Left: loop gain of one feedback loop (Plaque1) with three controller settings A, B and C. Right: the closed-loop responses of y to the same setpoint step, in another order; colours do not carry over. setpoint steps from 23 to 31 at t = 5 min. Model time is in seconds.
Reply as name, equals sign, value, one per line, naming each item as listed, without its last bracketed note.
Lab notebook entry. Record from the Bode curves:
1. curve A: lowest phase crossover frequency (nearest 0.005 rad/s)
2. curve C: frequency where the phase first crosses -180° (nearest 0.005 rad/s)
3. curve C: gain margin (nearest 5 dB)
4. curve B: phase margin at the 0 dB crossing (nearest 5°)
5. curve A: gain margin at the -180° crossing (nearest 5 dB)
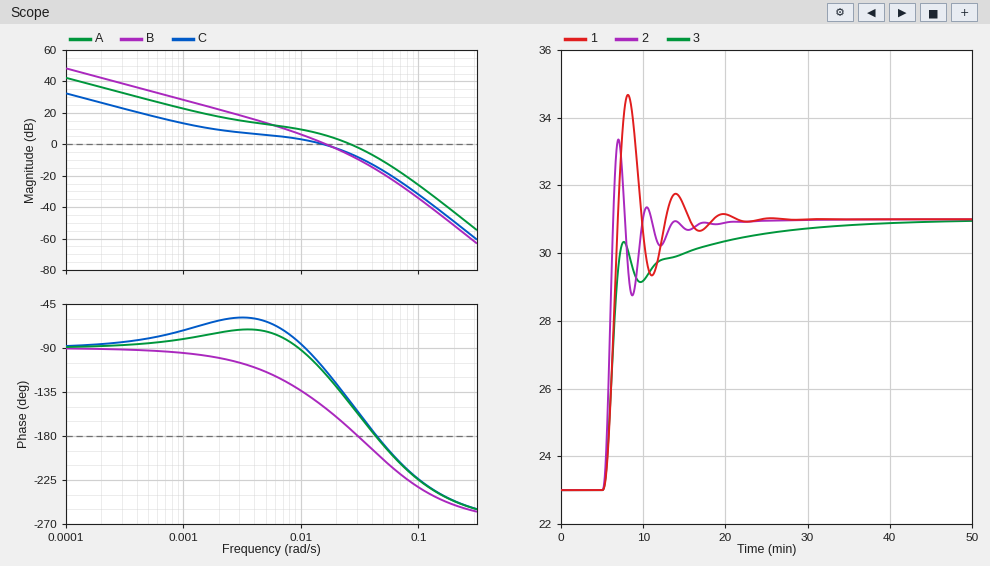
curve A: lowest phase crossover frequency = 0.045 rad/s
curve C: frequency where the phase first crosses -180° = 0.045 rad/s
curve C: gain margin = 15 dB
curve B: phase margin at the 0 dB crossing = 30°
curve A: gain margin at the -180° crossing = 10 dB
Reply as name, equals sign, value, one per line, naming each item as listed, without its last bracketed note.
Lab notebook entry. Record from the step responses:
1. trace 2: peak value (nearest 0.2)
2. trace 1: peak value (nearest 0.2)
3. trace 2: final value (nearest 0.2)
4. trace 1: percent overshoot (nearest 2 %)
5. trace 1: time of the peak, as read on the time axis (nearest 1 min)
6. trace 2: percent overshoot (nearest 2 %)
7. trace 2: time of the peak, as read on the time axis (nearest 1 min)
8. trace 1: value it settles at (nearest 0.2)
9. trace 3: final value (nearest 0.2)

trace 2: peak value = 33.4
trace 1: peak value = 34.6
trace 2: final value = 31.0
trace 1: percent overshoot = 46 %
trace 1: time of the peak, as read on the time axis = 8 min
trace 2: percent overshoot = 30 %
trace 2: time of the peak, as read on the time axis = 7 min
trace 1: value it settles at = 31.0
trace 3: final value = 31.0
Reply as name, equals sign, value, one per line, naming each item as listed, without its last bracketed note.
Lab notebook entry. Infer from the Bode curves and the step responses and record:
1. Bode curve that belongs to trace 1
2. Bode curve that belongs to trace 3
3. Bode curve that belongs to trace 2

Bode curve that belongs to trace 1 = B
Bode curve that belongs to trace 3 = C
Bode curve that belongs to trace 2 = A
